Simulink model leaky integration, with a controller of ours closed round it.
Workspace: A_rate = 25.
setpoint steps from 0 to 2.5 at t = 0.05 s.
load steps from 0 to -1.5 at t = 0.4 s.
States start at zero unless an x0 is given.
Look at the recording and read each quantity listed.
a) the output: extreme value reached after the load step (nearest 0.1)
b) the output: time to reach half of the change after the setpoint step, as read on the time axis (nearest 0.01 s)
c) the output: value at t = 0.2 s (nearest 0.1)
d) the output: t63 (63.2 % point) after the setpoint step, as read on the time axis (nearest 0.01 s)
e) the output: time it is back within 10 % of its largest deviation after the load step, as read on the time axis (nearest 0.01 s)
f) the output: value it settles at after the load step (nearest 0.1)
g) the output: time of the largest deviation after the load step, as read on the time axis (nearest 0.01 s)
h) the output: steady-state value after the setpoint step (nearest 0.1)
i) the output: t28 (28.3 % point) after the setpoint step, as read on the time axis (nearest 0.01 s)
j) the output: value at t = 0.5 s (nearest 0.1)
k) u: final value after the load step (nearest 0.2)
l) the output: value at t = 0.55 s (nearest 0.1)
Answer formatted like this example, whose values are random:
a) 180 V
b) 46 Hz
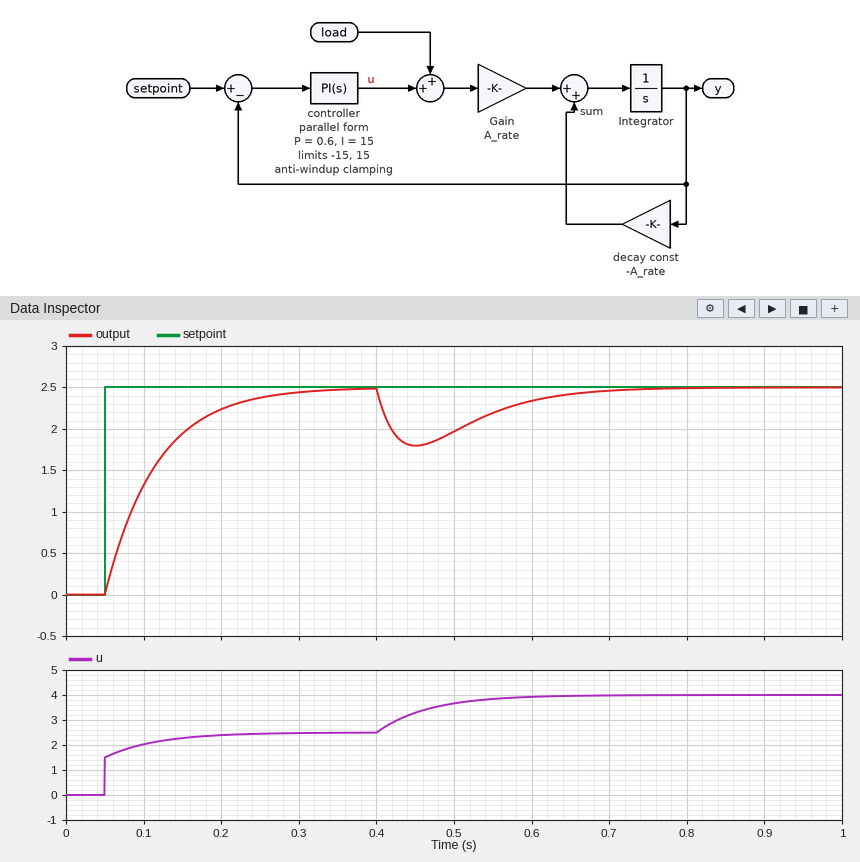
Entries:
a) 1.8
b) 0.10 s
c) 2.2
d) 0.12 s
e) 0.66 s
f) 2.5
g) 0.45 s
h) 2.5
i) 0.07 s
j) 2.0
k) 4.0
l) 2.2
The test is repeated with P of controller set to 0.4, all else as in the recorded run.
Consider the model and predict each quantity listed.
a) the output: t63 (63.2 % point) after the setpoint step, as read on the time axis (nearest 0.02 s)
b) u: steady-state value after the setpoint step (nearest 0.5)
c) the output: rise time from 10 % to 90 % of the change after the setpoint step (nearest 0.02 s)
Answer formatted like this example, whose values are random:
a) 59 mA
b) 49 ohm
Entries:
a) 0.12 s
b) 2.5
c) 0.14 s
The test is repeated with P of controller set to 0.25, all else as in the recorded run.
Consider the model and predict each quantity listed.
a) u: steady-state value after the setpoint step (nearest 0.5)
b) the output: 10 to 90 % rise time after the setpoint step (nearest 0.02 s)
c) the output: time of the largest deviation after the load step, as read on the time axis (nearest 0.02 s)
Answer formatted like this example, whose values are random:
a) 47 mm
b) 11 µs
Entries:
a) 2.5
b) 0.12 s
c) 0.46 s
